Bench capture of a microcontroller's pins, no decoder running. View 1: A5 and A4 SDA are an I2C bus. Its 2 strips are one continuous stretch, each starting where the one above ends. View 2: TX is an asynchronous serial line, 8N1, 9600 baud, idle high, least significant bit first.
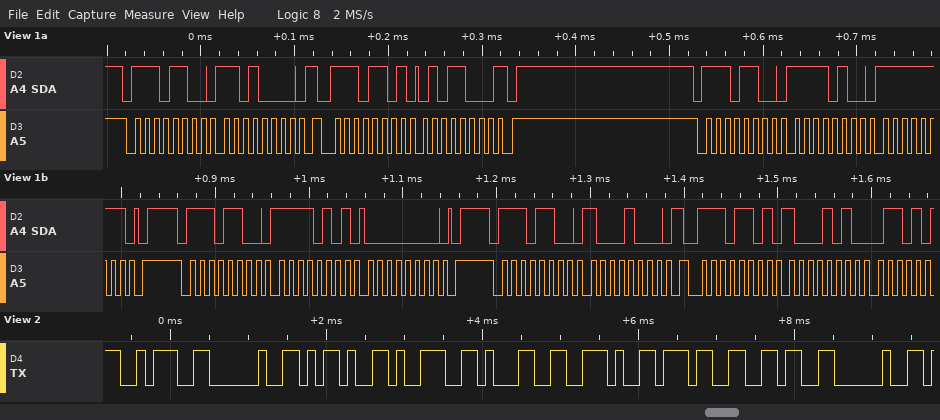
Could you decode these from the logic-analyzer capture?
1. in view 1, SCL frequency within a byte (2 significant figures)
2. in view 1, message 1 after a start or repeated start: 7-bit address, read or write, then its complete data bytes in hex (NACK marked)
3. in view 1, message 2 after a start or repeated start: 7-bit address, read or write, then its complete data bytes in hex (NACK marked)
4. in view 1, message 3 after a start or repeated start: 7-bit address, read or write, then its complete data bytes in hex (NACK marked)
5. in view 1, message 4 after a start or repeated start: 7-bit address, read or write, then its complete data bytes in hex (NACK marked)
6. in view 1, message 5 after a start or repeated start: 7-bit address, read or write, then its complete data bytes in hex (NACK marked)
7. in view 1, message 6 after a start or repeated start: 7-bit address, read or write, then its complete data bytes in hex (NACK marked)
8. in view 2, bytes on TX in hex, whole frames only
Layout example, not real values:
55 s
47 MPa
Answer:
100 kHz
0x76 write: D0
0x76 read: 58 NACK
0x76 write: F4 FF
0x76 write: F5 00
0x76 write: 88
0x76 read: 8A
3A 20 2D 39 31 2E 37 36 20
